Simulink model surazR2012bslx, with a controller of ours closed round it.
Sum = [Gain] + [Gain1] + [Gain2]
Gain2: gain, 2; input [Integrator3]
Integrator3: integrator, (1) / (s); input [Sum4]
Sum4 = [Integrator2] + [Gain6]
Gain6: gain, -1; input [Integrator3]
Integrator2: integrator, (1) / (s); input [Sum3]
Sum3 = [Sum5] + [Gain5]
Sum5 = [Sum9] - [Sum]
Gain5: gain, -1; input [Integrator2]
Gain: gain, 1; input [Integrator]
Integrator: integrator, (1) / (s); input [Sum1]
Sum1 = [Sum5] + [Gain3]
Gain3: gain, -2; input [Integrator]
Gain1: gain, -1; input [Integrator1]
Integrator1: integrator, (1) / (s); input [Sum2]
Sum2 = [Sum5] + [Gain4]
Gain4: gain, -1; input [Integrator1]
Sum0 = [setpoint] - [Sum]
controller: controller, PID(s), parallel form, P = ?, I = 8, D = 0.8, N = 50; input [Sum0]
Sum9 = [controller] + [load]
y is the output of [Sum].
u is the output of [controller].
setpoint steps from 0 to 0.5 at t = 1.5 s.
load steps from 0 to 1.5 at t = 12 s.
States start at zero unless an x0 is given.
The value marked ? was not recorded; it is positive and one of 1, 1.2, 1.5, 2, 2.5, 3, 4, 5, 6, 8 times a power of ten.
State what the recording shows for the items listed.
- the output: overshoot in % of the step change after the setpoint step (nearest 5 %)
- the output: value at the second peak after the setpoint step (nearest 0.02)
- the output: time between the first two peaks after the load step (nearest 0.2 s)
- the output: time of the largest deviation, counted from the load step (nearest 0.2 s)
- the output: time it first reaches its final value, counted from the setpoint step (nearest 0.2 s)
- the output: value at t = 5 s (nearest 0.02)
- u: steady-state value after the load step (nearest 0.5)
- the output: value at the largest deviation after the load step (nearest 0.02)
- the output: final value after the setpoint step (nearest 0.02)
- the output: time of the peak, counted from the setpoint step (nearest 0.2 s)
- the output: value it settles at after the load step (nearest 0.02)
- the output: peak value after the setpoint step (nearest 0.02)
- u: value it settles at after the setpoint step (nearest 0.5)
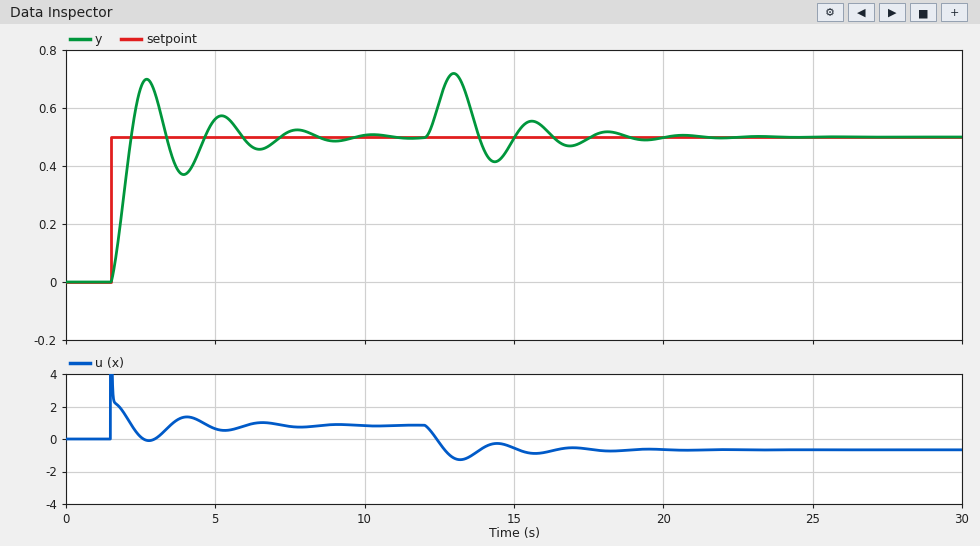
40 %
0.58
2.6 s
1.0 s
0.6 s
0.56
-0.5
0.72
0.50
1.2 s
0.50
0.70
1.0
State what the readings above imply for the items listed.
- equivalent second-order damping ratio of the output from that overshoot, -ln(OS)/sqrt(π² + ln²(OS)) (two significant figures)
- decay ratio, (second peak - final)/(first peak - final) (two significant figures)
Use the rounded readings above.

0.28
0.40
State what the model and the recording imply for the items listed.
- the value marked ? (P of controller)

5
